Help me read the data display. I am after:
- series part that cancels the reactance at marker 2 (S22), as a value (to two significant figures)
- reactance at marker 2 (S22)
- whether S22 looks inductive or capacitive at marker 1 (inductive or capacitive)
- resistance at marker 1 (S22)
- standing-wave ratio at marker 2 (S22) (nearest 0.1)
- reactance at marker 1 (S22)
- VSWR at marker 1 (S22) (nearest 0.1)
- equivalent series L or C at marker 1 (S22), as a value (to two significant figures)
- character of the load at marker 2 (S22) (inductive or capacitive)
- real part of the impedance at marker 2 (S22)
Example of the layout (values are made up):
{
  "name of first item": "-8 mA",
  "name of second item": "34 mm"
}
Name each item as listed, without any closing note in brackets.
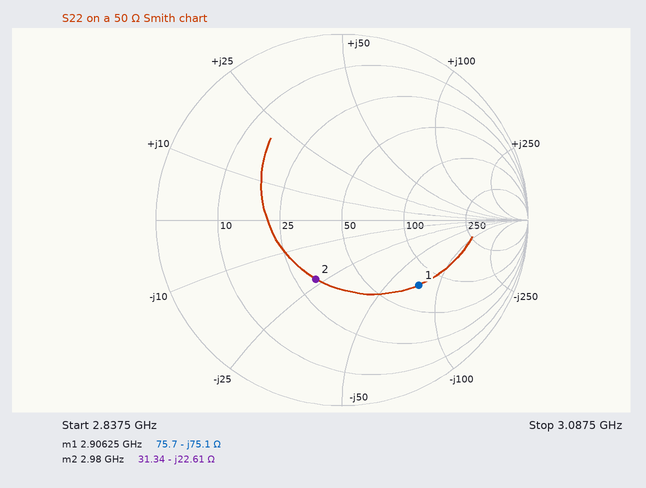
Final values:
{
  "series part that cancels the reactance at marker 2 (S22), as a value": "1.2 nH",
  "reactance at marker 2": "-22.61 Ω",
  "whether S22 looks inductive or capacitive at marker 1": "capacitive",
  "resistance at marker 1": "75.7 Ω",
  "standing-wave ratio at marker 2 (S22)": "2.1",
  "reactance at marker 1": "-75.1 Ω",
  "VSWR at marker 1 (S22)": "3.4",
  "equivalent series L or C at marker 1 (S22), as a value": "730 fF",
  "character of the load at marker 2 (S22)": "capacitive",
  "real part of the impedance at marker 2": "31.34 Ω"
}
